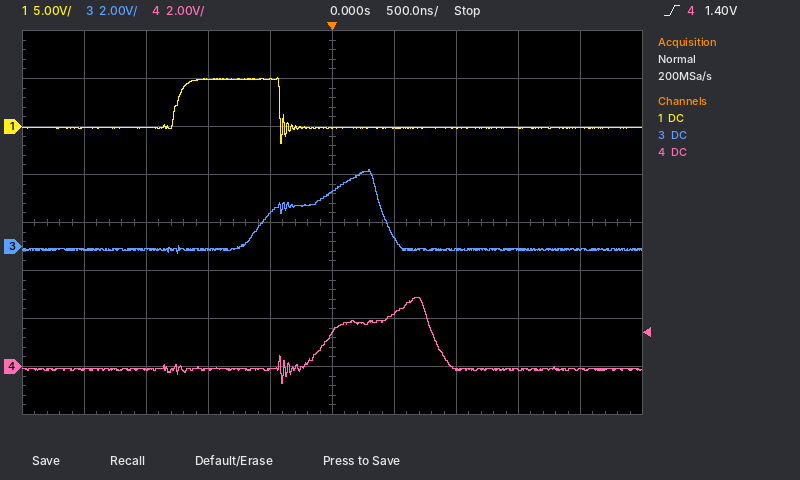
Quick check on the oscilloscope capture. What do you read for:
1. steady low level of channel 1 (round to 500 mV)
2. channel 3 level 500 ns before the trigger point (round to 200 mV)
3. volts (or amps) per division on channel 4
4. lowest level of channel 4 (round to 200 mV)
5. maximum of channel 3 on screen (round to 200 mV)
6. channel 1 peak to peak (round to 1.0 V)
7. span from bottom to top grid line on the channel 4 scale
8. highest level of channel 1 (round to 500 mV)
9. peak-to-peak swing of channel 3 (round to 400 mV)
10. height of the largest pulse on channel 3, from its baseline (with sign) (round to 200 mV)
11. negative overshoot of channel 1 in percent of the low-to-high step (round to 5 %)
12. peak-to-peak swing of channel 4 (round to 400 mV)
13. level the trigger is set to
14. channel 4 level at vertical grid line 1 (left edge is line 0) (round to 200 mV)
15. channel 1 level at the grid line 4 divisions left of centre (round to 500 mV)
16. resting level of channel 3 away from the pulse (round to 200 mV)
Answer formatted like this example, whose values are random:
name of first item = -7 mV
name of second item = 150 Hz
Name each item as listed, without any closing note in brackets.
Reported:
steady low level of channel 1 = 0.0 V
channel 3 level 500 ns before the trigger point = 1.4 V
volts (or amps) per division on channel 4 = 2 V
lowest level of channel 4 = -800 mV
maximum of channel 3 on screen = 3.2 V
channel 1 peak to peak = 7.0 V
span from bottom to top grid line on the channel 4 scale = 16 V
highest level of channel 1 = 5.0 V
peak-to-peak swing of channel 3 = 3.6 V
height of the largest pulse on channel 3, from its baseline (with sign) = +3.4 V
negative overshoot of channel 1 in percent of the low-to-high step = 35 %
peak-to-peak swing of channel 4 = 3.6 V
level the trigger is set to = 1.40 V
channel 4 level at vertical grid line 1 (left edge is line 0) = -200 mV
channel 1 level at the grid line 4 divisions left of centre = 0.0 V
resting level of channel 3 away from the pulse = -200 mV
